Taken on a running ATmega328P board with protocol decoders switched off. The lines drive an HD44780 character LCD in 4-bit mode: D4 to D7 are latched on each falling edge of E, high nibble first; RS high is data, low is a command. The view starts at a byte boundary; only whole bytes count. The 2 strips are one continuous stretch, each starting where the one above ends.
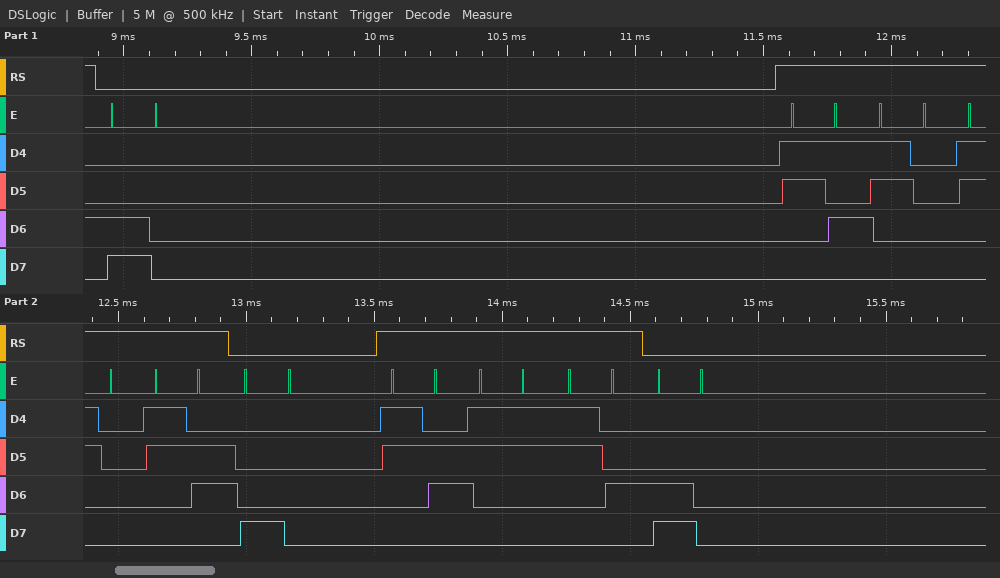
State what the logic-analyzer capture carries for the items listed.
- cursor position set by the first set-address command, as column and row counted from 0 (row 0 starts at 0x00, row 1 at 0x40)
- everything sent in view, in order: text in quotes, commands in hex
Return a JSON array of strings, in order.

["column 0, row 1", "0xC0 \"5006\" 0x80 \"634\" 0xC0"]
